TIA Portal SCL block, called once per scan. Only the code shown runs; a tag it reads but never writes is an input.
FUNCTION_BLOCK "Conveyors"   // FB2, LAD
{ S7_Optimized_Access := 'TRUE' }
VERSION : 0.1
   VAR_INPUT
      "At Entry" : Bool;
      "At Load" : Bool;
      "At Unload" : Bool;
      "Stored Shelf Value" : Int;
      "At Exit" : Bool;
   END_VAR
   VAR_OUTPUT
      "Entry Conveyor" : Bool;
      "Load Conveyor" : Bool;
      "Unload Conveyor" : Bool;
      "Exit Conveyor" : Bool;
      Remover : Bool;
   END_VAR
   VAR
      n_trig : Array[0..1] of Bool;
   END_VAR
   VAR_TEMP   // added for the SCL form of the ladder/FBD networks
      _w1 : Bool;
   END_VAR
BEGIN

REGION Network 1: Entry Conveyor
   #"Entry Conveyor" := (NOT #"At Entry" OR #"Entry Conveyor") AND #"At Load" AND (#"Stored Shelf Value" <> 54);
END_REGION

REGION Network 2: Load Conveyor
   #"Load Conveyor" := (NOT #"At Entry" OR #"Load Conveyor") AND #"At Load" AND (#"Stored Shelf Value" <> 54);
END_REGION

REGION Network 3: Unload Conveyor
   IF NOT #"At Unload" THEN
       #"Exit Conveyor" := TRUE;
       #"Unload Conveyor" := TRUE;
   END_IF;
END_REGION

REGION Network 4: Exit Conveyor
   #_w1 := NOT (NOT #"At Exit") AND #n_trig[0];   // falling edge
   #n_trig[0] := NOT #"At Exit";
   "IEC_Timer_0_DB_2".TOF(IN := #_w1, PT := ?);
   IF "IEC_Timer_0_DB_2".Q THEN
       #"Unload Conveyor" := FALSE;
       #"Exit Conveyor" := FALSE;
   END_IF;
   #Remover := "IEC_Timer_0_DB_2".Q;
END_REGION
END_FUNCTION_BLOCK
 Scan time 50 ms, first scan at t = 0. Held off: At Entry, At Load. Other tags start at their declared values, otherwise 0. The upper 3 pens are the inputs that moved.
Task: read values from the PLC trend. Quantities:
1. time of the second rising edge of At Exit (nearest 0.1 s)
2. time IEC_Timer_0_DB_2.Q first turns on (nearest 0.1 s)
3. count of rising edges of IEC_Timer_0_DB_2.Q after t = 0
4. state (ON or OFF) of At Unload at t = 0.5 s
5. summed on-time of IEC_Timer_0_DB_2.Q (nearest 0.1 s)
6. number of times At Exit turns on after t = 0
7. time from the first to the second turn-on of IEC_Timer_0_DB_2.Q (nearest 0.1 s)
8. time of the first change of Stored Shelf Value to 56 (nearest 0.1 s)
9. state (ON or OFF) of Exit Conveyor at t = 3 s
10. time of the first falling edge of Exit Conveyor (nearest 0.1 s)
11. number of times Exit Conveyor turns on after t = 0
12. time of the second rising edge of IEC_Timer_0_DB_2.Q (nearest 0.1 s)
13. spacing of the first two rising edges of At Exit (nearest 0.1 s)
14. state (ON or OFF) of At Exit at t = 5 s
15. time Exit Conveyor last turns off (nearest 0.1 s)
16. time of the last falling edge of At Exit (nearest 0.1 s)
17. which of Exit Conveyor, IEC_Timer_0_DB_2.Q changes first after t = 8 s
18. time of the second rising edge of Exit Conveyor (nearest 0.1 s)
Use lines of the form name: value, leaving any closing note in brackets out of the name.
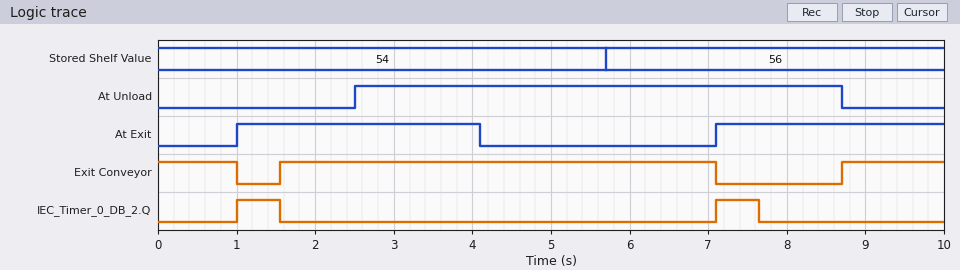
time of the second rising edge of At Exit: 7.1 s
time IEC_Timer_0_DB_2.Q first turns on: 1.0 s
count of rising edges of IEC_Timer_0_DB_2.Q after t = 0: 2
state (ON or OFF) of At Unload at t = 0.5 s: OFF
summed on-time of IEC_Timer_0_DB_2.Q: 1.1 s
number of times At Exit turns on after t = 0: 2
time from the first to the second turn-on of IEC_Timer_0_DB_2.Q: 6.1 s
time of the first change of Stored Shelf Value to 56: 5.7 s
state (ON or OFF) of Exit Conveyor at t = 3 s: ON
time of the first falling edge of Exit Conveyor: 1.0 s
number of times Exit Conveyor turns on after t = 0: 2
time of the second rising edge of IEC_Timer_0_DB_2.Q: 7.1 s
spacing of the first two rising edges of At Exit: 6.1 s
state (ON or OFF) of At Exit at t = 5 s: OFF
time Exit Conveyor last turns off: 7.1 s
time of the last falling edge of At Exit: 4.1 s
which of Exit Conveyor, IEC_Timer_0_DB_2.Q changes first after t = 8 s: Exit Conveyor
time of the second rising edge of Exit Conveyor: 8.7 s
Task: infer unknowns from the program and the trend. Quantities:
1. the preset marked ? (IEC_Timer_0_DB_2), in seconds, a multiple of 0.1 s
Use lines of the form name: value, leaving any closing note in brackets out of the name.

the preset marked ? (IEC_Timer_0_DB_2), in seconds, a multiple of 0.1 s: 0.5 s
